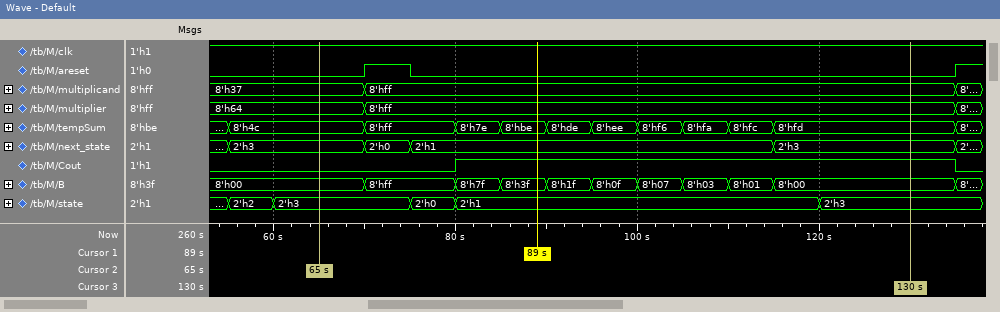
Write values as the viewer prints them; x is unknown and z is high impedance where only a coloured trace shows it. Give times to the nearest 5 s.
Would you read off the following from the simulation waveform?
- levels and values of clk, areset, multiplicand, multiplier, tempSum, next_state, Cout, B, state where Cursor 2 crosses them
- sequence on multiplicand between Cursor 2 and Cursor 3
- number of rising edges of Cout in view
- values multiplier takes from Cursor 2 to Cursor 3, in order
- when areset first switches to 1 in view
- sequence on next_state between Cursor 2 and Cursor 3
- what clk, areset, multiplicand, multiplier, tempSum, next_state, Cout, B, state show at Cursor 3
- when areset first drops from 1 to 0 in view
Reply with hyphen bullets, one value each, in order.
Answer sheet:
- clk=1, areset=0, multiplicand=8'h37, multiplier=8'h64, tempSum=8'h4c, next_state=2'h3, Cout=0, B=8'h00, state=2'h3
- 8'h37, 8'hff
- 1
- 8'h64, 8'hff
- 70 s
- 2'h3, 2'h0, 2'h1, 2'h3
- clk=1, areset=0, multiplicand=8'hff, multiplier=8'hff, tempSum=8'hfd, next_state=2'h3, Cout=1, B=8'h00, state=2'h3
- 75 s
